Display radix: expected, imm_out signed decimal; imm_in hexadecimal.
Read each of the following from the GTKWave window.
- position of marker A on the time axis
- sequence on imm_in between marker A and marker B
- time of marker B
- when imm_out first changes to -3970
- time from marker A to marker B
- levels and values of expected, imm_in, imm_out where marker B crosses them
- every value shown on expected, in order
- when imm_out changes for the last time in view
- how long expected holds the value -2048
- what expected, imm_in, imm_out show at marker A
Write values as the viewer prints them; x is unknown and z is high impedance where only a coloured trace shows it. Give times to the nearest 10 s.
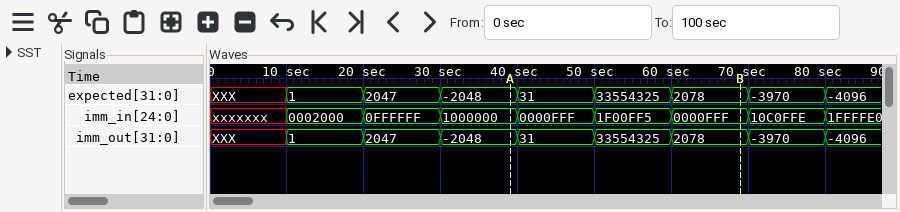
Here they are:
40 s
1000000, 0000FFF, 1F00FF5, 0000FFF
70 s
70 s
30 s
expected=2078, imm_in=0000FFF, imm_out=2078
XXX, 1, 2047, -2048, 31, 33554325, 2078, -3970, -4096
80 s
10 s
expected=-2048, imm_in=1000000, imm_out=-2048
